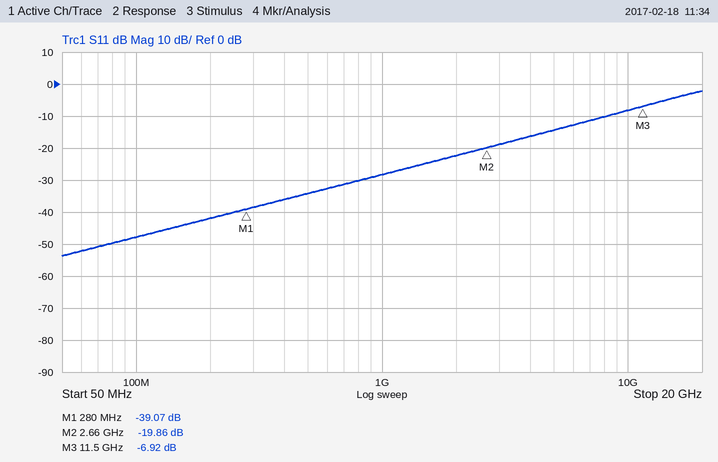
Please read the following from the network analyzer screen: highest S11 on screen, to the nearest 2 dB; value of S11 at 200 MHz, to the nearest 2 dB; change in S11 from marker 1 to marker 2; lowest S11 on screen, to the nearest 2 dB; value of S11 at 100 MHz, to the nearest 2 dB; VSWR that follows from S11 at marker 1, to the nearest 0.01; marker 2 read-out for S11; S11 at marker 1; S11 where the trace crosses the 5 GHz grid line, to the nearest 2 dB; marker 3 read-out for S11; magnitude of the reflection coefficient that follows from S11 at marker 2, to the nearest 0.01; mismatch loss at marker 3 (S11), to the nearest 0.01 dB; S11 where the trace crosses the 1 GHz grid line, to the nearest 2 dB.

-2 dB
-42 dB
19.21 dB
-54 dB
-48 dB
1.02
-19.86 dB
-39.07 dB
-14 dB
-6.92 dB
0.10
0.99 dB
-28 dB
